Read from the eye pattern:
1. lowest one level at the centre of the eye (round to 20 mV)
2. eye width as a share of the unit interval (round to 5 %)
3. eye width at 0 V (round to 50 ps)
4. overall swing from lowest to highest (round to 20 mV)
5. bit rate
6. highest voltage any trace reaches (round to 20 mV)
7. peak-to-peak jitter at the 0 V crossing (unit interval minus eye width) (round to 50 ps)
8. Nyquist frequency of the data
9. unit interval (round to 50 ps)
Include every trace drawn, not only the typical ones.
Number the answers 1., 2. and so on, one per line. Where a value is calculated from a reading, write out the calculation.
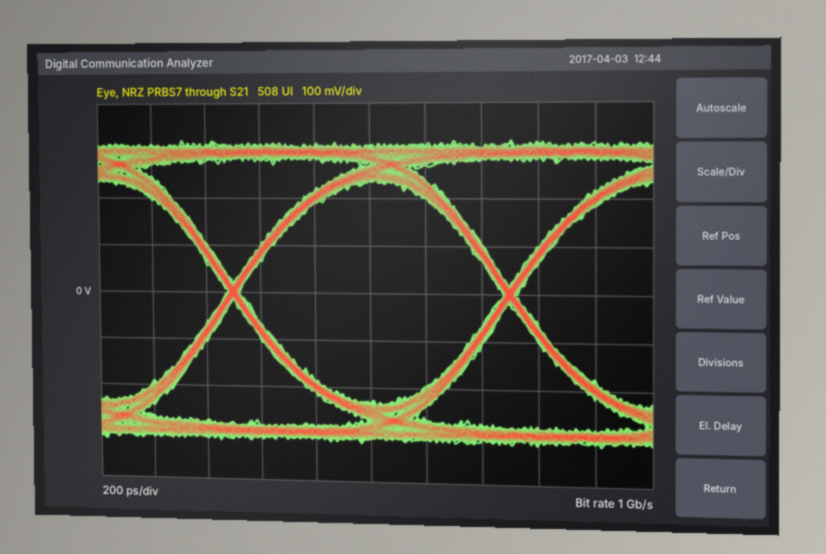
1. 240 mV
2. 950 ps / 1.00 ns ≈ 95 %
3. 950 ps
4. 640 mV
5. 1 Gb/s
6. 320 mV
7. 50 ps
8. 500 MHz
9. 1.00 ns
